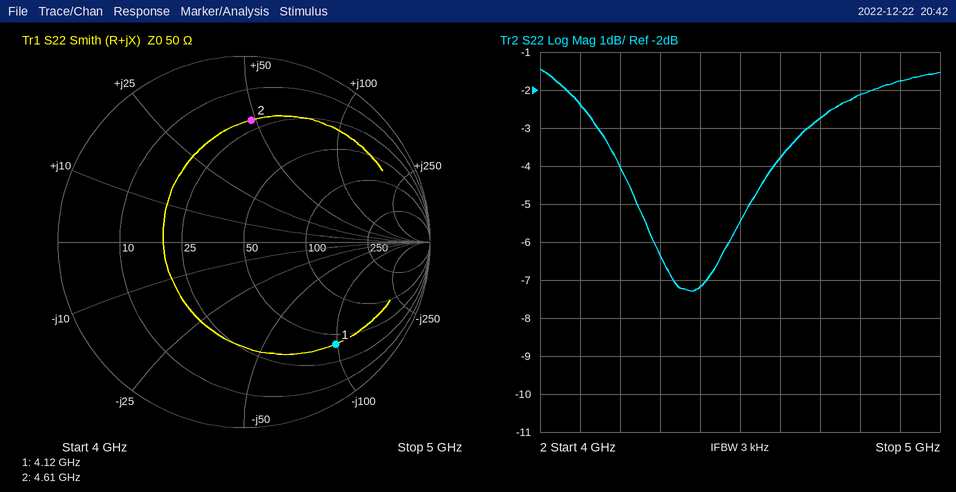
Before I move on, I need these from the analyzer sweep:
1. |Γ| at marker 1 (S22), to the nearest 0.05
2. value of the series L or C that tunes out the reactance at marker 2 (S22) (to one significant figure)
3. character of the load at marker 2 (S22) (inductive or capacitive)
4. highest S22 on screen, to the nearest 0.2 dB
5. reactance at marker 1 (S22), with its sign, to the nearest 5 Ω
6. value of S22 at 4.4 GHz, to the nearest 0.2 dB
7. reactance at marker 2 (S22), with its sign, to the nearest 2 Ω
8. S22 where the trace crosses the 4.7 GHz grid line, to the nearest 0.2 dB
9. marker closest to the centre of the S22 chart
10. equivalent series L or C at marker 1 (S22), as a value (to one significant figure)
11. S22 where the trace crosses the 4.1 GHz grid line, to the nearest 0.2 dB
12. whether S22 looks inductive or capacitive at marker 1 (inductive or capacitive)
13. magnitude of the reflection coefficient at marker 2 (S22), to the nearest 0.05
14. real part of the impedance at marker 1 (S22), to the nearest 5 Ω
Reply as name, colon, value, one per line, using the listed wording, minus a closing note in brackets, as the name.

|Γ| at marker 1 (S22), to the nearest 0.05: 0.75
value of the series L or C that tunes out the reactance at marker 2 (S22): 700 fF
character of the load at marker 2 (S22): inductive
highest S22 on screen, to the nearest 0.2 dB: -1.4 dB
reactance at marker 1 (S22), with its sign, to the nearest 5 Ω: -100 Ω
value of S22 at 4.4 GHz, to the nearest 0.2 dB: -7.2 dB
reactance at marker 2 (S22), with its sign, to the nearest 2 Ω: +48 Ω
S22 where the trace crosses the 4.7 GHz grid line, to the nearest 0.2 dB: -2.8 dB
marker closest to the centre of the S22 chart: marker 2
equivalent series L or C at marker 1 (S22), as a value: 400 fF
S22 where the trace crosses the 4.1 GHz grid line, to the nearest 0.2 dB: -2.4 dB
whether S22 looks inductive or capacitive at marker 1: capacitive
magnitude of the reflection coefficient at marker 2 (S22), to the nearest 0.05: 0.65
real part of the impedance at marker 1 (S22), to the nearest 5 Ω: 40 Ω
